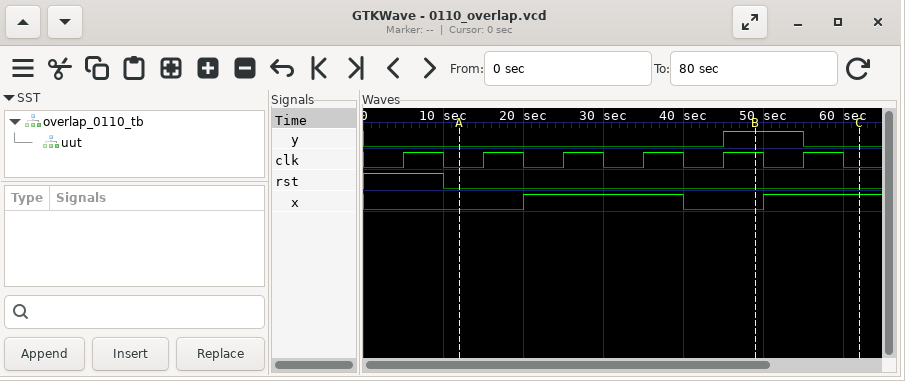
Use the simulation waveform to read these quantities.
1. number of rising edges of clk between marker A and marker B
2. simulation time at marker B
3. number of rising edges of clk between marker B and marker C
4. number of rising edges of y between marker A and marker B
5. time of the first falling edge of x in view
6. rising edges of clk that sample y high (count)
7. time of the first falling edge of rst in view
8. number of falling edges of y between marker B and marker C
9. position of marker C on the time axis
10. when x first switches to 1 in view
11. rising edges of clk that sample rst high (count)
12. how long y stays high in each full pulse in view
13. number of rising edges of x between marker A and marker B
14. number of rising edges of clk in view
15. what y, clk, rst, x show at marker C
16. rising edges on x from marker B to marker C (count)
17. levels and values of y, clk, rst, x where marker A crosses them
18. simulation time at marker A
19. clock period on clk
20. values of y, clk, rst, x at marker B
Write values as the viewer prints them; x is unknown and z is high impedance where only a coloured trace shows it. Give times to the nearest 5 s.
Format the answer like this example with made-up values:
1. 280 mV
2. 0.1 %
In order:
1. 4
2. 50 s
3. 1
4. 1
5. 40 s
6. 1
7. 10 s
8. 1
9. 60 s
10. 20 s
11. 1
12. 10 s
13. 1
14. 6
15. y=0, clk=0, rst=0, x=1
16. 1
17. y=0, clk=0, rst=0, x=0
18. 10 s
19. 10 s
20. y=1, clk=1, rst=0, x=0
